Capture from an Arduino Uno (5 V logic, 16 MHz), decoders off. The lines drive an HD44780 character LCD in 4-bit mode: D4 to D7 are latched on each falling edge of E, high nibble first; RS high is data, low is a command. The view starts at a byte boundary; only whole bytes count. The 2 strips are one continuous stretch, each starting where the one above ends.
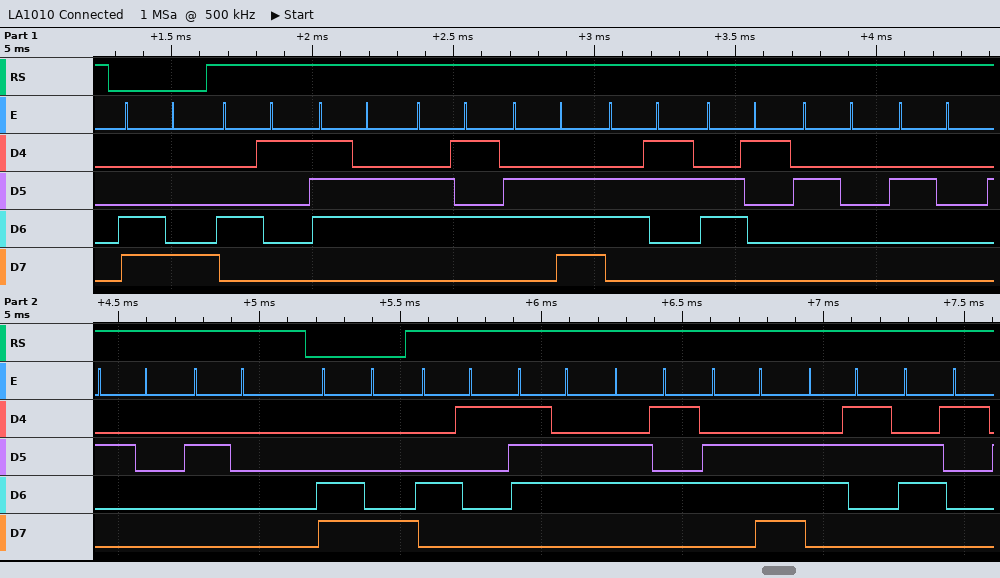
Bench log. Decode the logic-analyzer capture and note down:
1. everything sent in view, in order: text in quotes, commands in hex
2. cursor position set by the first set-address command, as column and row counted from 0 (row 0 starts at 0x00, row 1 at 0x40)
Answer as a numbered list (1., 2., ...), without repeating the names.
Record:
1. 0xC8 "Avenca    " 0xC8 "Avenca"
2. column 8, row 1
